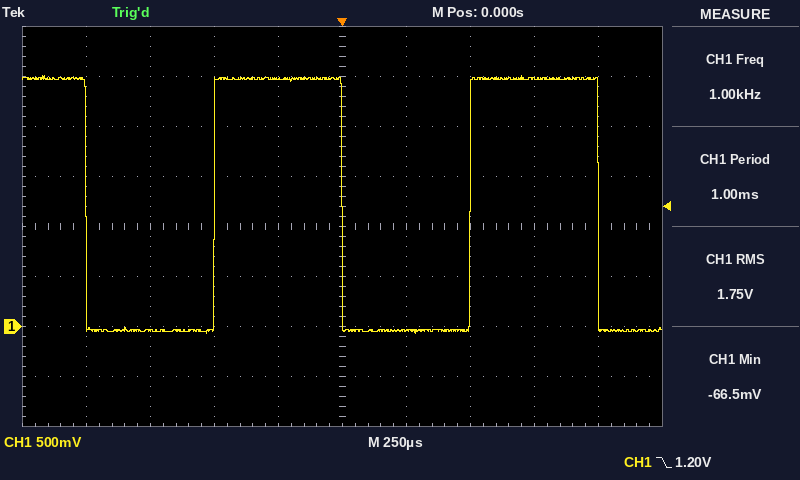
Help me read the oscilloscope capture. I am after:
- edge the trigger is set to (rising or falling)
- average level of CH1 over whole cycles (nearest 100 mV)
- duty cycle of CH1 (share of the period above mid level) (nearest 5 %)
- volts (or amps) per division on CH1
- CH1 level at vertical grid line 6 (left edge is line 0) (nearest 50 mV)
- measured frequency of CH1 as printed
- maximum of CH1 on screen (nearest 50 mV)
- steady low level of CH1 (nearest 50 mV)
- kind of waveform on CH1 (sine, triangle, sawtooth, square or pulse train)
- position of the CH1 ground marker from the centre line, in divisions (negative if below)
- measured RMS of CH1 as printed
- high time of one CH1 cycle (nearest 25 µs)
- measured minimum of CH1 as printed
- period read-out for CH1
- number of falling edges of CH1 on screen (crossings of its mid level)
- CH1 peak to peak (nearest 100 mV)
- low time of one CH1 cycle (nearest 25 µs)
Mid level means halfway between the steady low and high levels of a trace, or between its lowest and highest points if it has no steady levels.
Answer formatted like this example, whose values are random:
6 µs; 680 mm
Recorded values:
falling; 1.2 V; 50 %; 500 mV; -50 mV; 1.00 kHz; 2.50 V; -50 mV; square; -2.0 div; 1.75 V; 500 µs; -66.5 mV; 1.00 ms; 3; 2.60 V; 500 µs
